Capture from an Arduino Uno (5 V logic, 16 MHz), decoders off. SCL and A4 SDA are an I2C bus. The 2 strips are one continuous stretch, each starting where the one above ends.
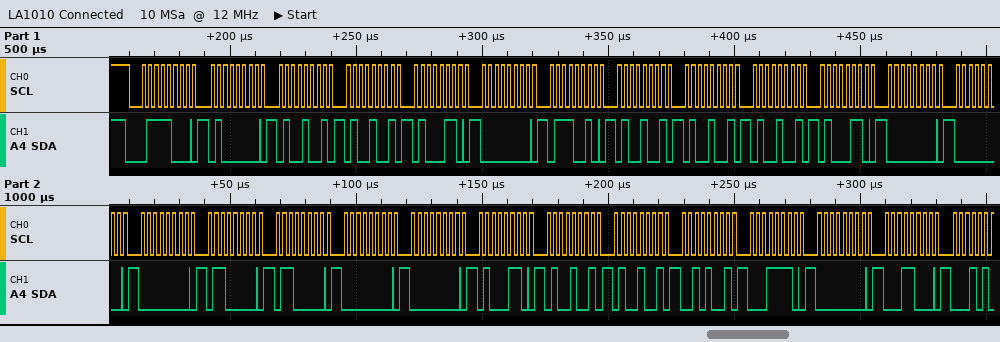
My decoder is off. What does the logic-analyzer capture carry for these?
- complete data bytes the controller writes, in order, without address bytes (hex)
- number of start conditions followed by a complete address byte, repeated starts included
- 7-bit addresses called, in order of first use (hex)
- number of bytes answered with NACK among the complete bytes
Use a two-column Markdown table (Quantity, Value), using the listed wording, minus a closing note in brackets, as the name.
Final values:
| Quantity | Value |
|---|---|
| complete data bytes the controller writes, in order, without address bytes | 40 49 49 46 00 72 49 49 49 46 00 00 00 60 60 00 00 46 49 49 29 1E 00 18 |
| number of start conditions followed by a complete address byte, repeated starts included | 1 |
| 7-bit addresses called, in order of first use | 0x3C |
| number of bytes answered with NACK among the complete bytes | 0 |
